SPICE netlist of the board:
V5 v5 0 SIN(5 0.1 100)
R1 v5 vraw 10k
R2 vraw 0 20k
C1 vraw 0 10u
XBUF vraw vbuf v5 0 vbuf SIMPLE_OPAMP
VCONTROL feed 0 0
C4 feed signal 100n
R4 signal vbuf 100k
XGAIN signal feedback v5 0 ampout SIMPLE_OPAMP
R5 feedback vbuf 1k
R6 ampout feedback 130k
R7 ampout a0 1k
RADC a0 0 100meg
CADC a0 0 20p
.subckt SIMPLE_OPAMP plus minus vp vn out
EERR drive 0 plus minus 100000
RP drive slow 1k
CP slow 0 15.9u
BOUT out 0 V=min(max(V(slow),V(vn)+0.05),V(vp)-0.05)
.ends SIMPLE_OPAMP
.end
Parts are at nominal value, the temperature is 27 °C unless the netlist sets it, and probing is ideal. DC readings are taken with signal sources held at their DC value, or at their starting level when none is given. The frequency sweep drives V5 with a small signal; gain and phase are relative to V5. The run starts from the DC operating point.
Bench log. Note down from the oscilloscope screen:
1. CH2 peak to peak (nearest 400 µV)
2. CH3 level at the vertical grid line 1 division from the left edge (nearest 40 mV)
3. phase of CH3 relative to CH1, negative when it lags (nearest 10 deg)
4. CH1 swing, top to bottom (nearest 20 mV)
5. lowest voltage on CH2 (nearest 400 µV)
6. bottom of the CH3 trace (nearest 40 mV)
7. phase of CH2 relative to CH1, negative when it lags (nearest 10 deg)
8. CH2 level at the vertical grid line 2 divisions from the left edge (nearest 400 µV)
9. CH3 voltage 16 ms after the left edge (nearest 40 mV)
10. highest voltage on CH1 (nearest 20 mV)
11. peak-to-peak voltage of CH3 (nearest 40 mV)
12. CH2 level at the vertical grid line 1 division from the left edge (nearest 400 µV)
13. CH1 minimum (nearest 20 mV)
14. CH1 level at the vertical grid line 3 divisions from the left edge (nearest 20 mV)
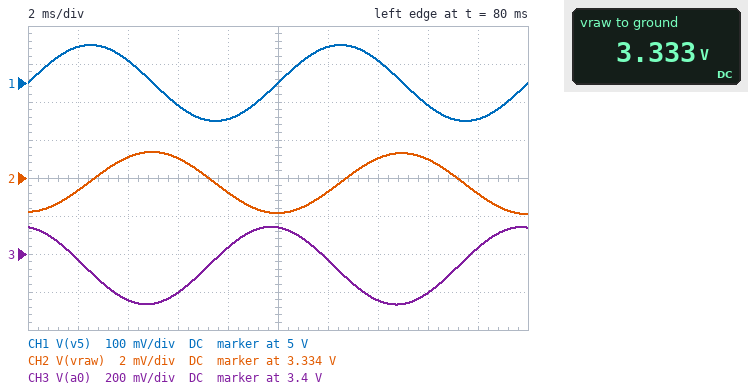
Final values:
3.2 mV
3.36 V
100 deg
200 mV
3.3320 V
3.12 V
-90 deg
3.3352 V
3.20 V
5.10 V
400 mV
3.3332 V
4.90 V
4.94 V
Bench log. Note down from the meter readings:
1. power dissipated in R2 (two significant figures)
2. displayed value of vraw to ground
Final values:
560 µW
3.333 V
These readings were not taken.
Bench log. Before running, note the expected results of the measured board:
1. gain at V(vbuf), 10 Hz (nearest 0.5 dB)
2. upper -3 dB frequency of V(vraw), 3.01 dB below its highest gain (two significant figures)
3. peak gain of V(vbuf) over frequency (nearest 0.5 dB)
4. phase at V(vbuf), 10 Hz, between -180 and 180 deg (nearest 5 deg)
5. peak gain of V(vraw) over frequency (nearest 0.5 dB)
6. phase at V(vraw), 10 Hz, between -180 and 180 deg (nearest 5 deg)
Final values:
-16.0 dB
2.4 Hz
-3.5 dB
-75 deg
-3.5 dB
-75 deg
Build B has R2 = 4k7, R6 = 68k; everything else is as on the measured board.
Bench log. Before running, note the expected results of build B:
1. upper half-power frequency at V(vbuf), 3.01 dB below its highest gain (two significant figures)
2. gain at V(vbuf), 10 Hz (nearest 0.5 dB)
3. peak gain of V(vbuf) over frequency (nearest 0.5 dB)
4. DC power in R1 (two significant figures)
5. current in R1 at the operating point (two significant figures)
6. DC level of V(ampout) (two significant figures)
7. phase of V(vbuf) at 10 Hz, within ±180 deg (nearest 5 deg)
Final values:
5.0 Hz
-17.0 dB
-10.0 dB
1.2 mW
340 µA
1.6 V
-65 deg
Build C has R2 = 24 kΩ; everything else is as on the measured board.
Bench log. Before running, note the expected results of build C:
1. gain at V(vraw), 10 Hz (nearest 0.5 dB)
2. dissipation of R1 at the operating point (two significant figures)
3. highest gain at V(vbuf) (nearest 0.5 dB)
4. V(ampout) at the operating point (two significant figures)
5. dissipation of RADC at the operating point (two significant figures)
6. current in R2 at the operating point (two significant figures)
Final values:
-16.0 dB
220 µW
-3.0 dB
3.5 V
120 nW
150 µA
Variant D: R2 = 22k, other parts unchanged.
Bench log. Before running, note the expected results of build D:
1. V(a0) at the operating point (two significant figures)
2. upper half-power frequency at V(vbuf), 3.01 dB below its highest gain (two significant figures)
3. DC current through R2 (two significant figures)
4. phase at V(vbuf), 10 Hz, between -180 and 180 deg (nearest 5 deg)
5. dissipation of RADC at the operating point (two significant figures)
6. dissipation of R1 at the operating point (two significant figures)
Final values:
3.4 V
2.3 Hz
160 µA
-75 deg
120 nW
240 µW
